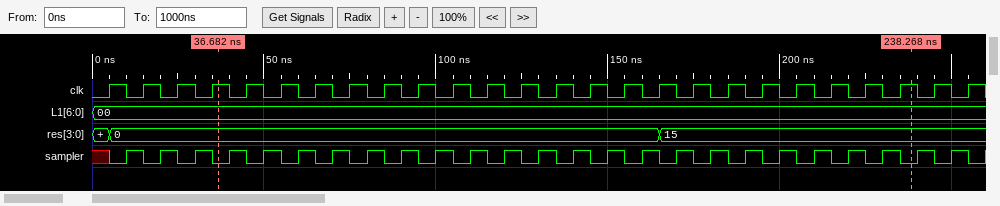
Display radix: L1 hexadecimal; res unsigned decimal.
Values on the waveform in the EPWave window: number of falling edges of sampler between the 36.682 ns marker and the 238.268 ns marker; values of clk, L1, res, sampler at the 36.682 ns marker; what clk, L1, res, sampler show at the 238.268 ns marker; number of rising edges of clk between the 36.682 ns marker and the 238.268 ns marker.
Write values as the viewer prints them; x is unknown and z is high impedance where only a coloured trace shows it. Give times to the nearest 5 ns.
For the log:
20
clk=1, L1=00, res=0, sampler=0
clk=1, L1=00, res=15, sampler=0
20
